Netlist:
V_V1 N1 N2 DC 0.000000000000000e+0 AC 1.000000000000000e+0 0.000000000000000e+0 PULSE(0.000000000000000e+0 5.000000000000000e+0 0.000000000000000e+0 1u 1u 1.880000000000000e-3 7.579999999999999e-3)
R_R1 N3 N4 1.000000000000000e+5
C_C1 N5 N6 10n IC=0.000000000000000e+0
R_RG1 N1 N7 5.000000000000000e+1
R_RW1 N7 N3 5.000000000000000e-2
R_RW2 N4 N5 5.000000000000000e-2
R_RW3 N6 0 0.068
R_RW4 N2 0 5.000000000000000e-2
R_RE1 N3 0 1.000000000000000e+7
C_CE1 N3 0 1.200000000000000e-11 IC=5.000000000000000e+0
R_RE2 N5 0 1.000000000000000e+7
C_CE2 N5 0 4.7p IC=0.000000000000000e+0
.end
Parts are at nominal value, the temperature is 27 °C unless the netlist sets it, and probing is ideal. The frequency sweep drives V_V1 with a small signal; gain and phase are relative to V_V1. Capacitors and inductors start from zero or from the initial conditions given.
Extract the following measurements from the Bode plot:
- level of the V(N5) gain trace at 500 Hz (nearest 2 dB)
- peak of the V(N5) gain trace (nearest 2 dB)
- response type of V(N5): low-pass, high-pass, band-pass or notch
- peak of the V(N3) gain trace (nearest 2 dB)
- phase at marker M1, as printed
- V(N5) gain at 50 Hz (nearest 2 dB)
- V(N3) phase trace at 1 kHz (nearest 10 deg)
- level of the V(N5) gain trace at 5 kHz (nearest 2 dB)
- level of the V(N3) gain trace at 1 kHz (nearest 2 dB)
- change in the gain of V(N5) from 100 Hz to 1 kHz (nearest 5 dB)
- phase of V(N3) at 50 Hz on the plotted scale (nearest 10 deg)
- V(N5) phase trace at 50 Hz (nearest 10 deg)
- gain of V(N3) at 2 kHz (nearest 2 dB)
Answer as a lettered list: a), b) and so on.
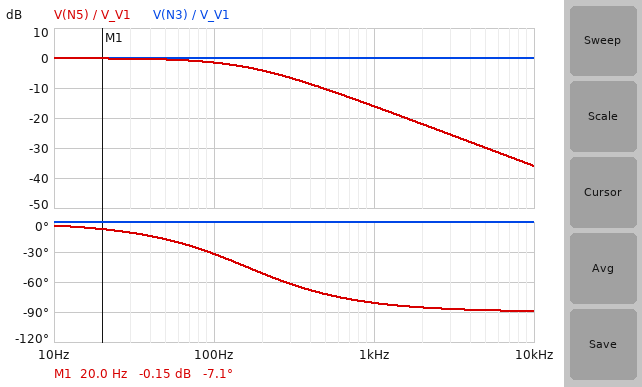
a) -10 dB
b) 0 dB
c) low-pass
d) 0 dB
e) -7.1 deg
f) 0 dB
g) 0 deg
h) -30 dB
i) 0 dB
j) -15 dB
k) 0 deg
l) -20 deg
m) 0 dB
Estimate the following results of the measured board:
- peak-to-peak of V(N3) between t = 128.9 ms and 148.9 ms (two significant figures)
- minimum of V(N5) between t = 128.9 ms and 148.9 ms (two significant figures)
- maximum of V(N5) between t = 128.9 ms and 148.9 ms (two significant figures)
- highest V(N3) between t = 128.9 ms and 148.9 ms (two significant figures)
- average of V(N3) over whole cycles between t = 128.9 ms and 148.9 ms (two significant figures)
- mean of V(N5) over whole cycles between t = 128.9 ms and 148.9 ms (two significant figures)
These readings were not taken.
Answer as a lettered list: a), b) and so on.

a) 5.0 V
b) 13 mV
c) 4.2 V
d) 5.0 V
e) 1.2 V
f) 1.2 V
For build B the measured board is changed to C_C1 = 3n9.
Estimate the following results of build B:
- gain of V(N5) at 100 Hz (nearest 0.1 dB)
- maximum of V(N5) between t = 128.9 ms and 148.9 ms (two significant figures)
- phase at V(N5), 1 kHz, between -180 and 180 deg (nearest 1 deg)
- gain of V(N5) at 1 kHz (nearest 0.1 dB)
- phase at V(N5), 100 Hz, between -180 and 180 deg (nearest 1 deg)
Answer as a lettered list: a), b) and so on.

a) -0.3 dB
b) 4.9 V
c) -68 deg
d) -8.5 dB
e) -14 deg
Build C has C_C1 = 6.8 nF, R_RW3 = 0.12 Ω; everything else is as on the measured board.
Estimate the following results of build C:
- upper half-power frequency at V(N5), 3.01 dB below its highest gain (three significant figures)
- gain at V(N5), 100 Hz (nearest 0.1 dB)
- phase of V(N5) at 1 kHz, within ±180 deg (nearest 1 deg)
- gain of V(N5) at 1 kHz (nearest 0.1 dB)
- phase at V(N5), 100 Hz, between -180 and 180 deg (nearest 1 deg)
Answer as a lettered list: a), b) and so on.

a) 236 Hz
b) -0.8 dB
c) -77 deg
d) -12.9 dB
e) -23 deg
